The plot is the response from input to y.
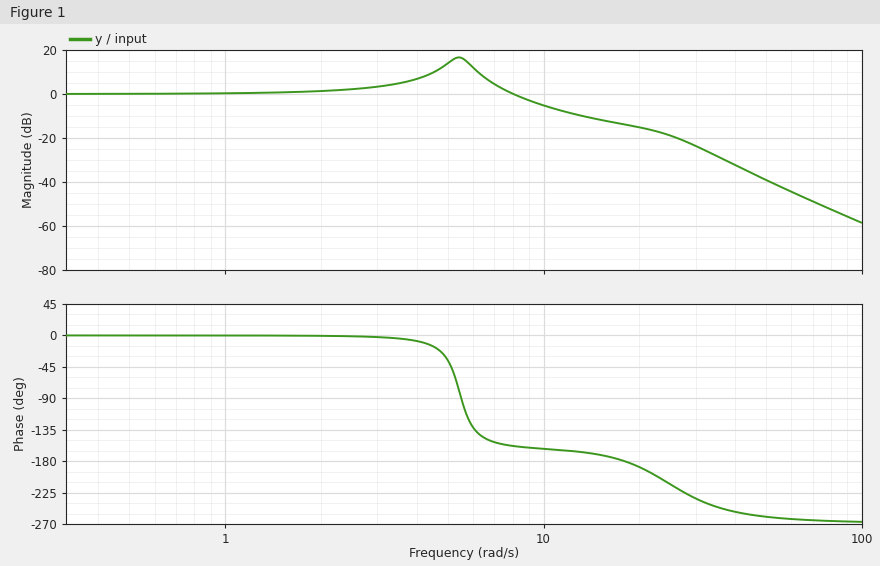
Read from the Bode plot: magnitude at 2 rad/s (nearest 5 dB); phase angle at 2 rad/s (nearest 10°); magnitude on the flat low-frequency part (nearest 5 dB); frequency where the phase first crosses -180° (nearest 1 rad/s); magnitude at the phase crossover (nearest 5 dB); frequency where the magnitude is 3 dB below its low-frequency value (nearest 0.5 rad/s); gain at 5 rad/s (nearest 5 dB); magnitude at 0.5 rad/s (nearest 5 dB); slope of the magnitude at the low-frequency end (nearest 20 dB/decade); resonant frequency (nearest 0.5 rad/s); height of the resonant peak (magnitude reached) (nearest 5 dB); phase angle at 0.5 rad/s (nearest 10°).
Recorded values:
0 dB
0°
0 dB
18 rad/s
-15 dB
9.0 rad/s
15 dB
0 dB
0 dB/decade
5.5 rad/s
15 dB
0°
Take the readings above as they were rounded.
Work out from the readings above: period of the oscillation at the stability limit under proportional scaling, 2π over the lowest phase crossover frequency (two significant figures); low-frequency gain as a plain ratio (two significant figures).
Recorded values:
0.35 s
1.0
